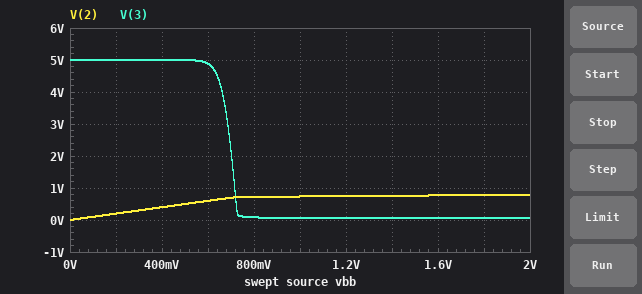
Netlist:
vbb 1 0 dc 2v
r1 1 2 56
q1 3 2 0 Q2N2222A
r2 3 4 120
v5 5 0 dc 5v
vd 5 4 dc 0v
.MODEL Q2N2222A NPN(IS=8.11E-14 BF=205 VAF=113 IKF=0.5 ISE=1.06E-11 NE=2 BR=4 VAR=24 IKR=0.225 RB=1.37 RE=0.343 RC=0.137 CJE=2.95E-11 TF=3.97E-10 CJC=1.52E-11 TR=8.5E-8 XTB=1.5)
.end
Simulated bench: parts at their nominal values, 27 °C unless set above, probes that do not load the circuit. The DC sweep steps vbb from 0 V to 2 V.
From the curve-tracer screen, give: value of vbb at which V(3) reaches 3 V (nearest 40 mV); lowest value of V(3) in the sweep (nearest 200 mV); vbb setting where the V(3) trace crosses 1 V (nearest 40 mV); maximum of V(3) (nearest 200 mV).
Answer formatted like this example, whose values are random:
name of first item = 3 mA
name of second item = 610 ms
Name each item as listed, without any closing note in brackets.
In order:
value of vbb at which V(3) reaches 3 V = 680 mV
lowest value of V(3) in the sweep = 0 V
vbb setting where the V(3) trace crosses 1 V = 720 mV
maximum of V(3) = 5.0 V
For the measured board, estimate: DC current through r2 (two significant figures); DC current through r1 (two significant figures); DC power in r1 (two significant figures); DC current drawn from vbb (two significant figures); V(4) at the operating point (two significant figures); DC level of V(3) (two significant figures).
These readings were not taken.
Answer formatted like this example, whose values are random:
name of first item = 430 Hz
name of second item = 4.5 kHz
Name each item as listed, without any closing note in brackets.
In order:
DC current through r2 = 41 mA
DC current through r1 = 22 mA
DC power in r1 = 26 mW
DC current drawn from vbb = 22 mA
V(4) at the operating point = 5.0 V
DC level of V(3) = 47 mV
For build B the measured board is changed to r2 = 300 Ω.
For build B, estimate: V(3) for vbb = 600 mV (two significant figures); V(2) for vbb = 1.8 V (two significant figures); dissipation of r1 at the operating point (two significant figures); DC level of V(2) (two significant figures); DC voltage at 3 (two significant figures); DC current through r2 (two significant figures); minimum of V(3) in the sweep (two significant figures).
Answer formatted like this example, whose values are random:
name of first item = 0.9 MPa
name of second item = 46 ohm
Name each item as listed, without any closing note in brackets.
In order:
V(3) for vbb = 600 mV = 4.7 V
V(2) for vbb = 1.8 V = 760 mV
dissipation of r1 at the operating point = 27 mW
DC level of V(2) = 770 mV
DC voltage at 3 = 29 mV
DC current through r2 = 17 mA
minimum of V(3) in the sweep = 27 mV
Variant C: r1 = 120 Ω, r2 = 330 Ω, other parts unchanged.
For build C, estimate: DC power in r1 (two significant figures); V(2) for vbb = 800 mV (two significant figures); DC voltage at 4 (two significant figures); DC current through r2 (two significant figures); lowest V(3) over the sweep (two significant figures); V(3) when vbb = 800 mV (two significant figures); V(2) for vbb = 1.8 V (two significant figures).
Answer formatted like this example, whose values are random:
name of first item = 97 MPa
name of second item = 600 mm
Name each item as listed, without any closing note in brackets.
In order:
DC power in r1 = 13 mW
V(2) for vbb = 800 mV = 690 mV
DC voltage at 4 = 5.0 V
DC current through r2 = 15 mA
lowest V(3) over the sweep = 26 mV
V(3) when vbb = 800 mV = 54 mV
V(2) for vbb = 1.8 V = 730 mV
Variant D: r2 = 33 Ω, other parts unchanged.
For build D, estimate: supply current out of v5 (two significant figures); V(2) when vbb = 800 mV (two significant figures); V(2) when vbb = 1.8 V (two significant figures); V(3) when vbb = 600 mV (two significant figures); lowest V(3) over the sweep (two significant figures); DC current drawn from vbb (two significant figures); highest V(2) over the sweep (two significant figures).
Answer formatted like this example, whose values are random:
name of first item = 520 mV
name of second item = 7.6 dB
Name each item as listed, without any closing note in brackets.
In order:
supply current out of v5 = 150 mA
V(2) when vbb = 800 mV = 760 mV
V(2) when vbb = 1.8 V = 830 mV
V(3) when vbb = 600 mV = 5.0 V
lowest V(3) over the sweep = 120 mV
DC current drawn from vbb = 21 mA
highest V(2) over the sweep = 840 mV
